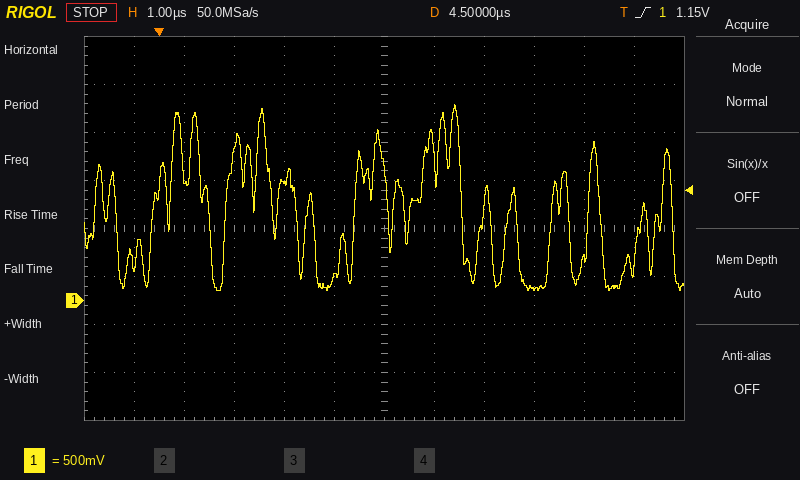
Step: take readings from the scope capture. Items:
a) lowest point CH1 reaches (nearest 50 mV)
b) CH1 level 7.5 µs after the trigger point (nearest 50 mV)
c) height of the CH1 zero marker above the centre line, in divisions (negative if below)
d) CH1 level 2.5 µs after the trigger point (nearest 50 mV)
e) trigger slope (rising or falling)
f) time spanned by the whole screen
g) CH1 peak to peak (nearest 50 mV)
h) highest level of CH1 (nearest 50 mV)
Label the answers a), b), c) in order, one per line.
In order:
a) 100 mV
b) 100 mV
c) -1.5 div
d) 1.25 V
e) rising
f) 12 µs
g) 1.95 V
h) 2.05 V
